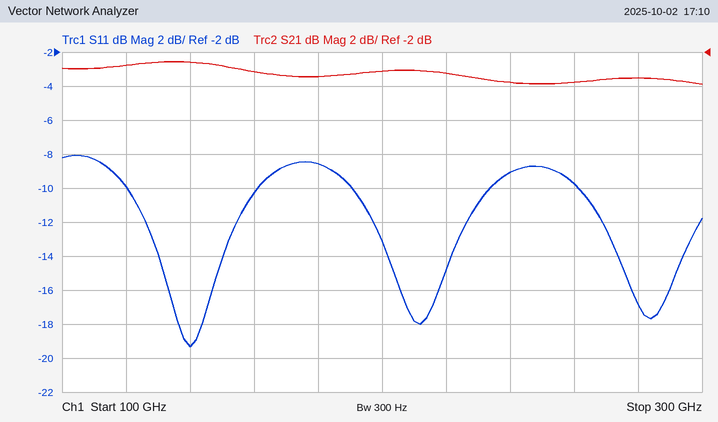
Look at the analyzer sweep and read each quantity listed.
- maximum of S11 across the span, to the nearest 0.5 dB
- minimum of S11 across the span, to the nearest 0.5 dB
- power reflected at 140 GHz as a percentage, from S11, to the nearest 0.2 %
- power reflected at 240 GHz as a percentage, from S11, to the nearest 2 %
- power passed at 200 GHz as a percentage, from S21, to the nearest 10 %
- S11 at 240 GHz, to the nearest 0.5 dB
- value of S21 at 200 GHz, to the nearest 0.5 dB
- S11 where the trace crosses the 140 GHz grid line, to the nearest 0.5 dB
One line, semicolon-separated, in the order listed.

-8.0 dB; -19.5 dB; 1.2 %; 12 %; 50 %; -9.0 dB; -3.0 dB; -19.5 dB
